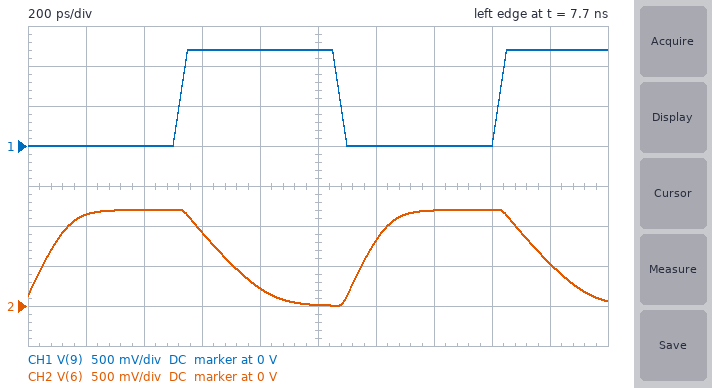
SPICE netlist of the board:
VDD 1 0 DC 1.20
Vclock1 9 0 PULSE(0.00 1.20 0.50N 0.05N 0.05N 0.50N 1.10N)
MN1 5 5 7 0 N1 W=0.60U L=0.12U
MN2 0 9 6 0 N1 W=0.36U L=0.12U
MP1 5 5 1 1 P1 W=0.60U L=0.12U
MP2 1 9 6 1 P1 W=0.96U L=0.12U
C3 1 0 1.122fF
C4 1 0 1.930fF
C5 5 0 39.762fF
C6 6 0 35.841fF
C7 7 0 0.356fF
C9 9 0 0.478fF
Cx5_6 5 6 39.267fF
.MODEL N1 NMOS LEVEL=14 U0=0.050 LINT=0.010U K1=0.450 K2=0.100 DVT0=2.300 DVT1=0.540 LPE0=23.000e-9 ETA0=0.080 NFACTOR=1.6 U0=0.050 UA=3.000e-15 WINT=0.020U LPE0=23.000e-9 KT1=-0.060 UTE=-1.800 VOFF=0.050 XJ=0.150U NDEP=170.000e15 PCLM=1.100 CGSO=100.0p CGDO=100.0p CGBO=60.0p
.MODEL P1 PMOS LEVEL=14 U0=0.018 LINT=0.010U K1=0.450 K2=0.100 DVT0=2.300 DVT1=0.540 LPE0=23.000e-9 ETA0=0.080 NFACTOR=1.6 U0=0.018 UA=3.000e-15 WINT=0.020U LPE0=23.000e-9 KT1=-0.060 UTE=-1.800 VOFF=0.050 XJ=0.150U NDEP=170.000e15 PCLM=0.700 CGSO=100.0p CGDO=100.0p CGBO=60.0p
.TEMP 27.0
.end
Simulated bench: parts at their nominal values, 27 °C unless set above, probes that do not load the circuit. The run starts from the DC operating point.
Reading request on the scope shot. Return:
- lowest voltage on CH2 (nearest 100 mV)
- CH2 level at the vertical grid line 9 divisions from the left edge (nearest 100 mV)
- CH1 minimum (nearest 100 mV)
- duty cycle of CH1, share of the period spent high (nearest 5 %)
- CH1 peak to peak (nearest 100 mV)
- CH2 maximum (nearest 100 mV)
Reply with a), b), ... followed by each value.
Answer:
a) 0 V
b) 500 mV
c) 0 V
d) 50 %
e) 1.2 V
f) 1.2 V
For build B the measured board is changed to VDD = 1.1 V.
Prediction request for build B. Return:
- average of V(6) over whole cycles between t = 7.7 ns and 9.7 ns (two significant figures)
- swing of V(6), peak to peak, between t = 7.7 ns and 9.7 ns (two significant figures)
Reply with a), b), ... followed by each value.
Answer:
a) 600 mV
b) 1.1 V
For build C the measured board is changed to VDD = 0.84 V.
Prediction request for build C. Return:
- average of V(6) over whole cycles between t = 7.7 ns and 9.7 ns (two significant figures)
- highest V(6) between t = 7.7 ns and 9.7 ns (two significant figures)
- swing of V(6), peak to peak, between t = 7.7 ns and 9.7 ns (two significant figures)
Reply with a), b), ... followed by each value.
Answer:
a) 410 mV
b) 840 mV
c) 850 mV
